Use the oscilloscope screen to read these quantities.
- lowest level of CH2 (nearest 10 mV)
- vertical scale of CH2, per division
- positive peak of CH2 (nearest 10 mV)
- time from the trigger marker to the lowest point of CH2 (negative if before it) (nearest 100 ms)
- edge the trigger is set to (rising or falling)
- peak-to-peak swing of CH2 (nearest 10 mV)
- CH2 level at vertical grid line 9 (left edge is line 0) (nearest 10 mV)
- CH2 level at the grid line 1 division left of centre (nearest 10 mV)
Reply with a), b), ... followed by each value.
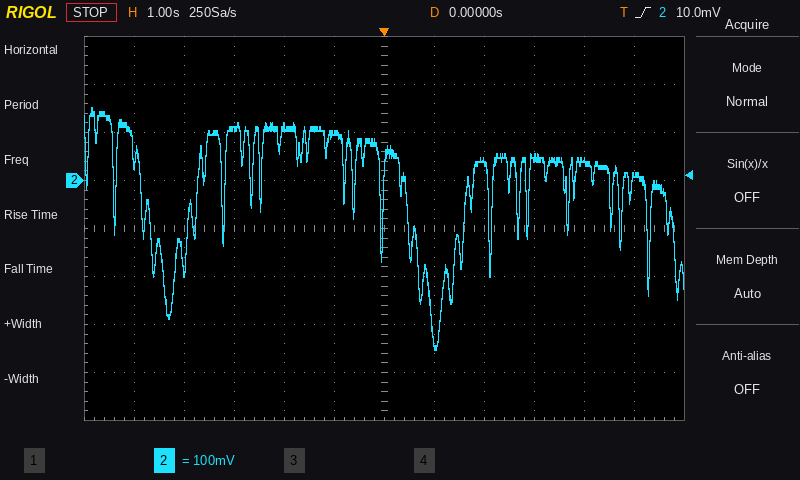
a) -350 mV
b) 100 mV
c) 150 mV
d) +1.0 s
e) rising
f) 500 mV
g) 50 mV
h) 100 mV
